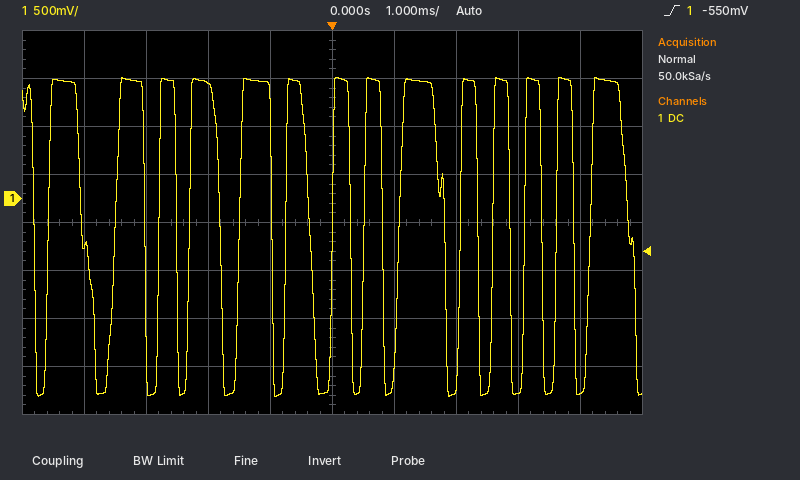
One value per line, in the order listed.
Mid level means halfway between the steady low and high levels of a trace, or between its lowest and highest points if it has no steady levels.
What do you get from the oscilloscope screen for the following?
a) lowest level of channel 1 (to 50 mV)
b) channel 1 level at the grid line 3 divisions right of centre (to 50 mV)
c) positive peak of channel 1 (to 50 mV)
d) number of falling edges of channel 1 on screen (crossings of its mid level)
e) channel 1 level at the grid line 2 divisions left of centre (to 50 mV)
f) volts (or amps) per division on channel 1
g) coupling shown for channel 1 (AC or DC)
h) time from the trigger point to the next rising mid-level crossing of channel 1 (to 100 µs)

-2.05 V
-2.00 V
1.25 V
15
1.20 V
500 mV
DC
500 µs
